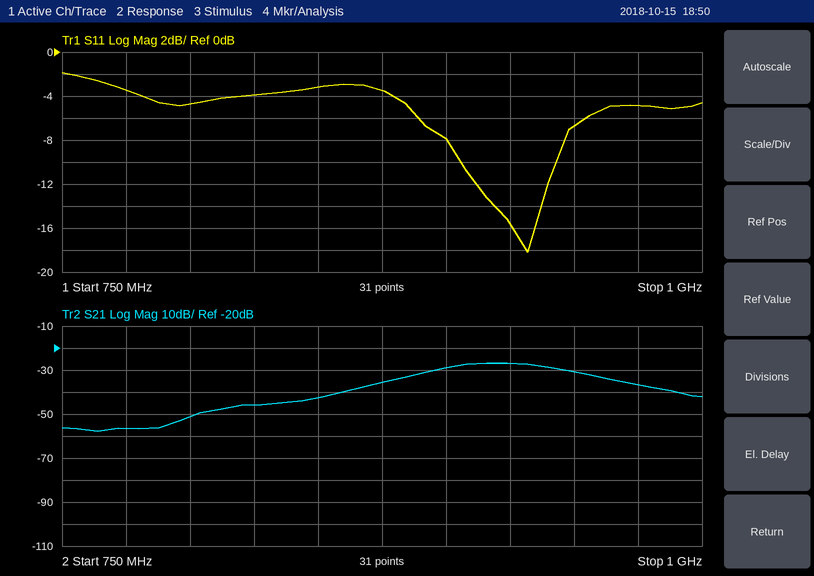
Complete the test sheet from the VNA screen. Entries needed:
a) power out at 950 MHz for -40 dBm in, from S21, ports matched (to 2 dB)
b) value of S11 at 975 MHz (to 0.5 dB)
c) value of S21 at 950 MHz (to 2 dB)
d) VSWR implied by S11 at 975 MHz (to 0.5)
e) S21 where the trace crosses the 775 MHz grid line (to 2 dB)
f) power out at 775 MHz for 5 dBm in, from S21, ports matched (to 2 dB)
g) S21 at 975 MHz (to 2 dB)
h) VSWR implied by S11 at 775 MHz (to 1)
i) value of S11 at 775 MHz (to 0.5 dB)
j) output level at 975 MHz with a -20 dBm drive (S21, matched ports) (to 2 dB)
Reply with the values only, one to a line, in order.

-70 dBm
-5.0 dB
-30 dB
3.5
-56 dB
-52 dBm
-36 dB
5
-3.5 dB
-56 dBm
